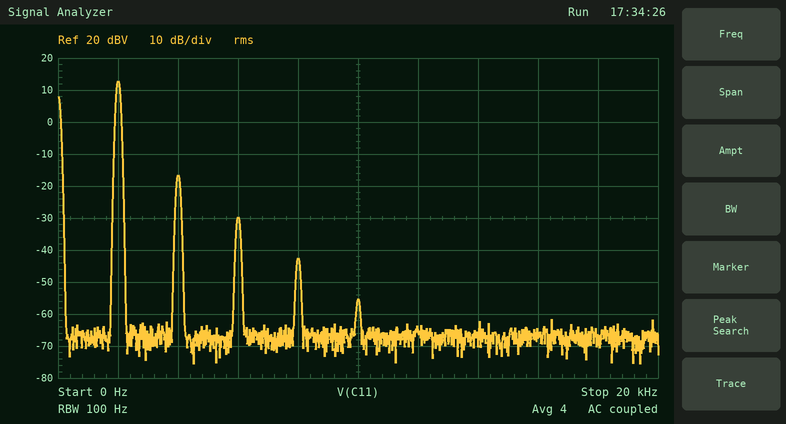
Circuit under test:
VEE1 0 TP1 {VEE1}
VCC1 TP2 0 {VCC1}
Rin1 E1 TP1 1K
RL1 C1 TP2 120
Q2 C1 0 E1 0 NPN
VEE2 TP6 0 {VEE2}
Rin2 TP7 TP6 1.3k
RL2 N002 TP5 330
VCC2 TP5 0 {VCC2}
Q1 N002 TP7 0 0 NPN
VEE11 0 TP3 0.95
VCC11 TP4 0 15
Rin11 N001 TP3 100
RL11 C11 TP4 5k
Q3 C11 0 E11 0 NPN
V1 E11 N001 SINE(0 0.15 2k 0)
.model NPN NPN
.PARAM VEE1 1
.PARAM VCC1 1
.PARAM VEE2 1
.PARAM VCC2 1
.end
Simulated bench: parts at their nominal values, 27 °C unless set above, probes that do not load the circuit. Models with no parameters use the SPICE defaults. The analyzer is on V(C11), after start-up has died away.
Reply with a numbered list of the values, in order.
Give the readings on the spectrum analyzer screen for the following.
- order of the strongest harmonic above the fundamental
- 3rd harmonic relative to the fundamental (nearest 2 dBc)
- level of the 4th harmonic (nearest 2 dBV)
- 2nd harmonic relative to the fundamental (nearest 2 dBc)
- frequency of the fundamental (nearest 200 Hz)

1. 2
2. -42 dBc
3. -42 dBV
4. -30 dBc
5. 2.0 kHz
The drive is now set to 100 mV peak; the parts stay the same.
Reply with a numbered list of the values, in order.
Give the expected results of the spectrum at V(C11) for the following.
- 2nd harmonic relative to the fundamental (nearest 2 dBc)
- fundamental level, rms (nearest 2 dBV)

1. -34 dBc
2. 10 dBV
